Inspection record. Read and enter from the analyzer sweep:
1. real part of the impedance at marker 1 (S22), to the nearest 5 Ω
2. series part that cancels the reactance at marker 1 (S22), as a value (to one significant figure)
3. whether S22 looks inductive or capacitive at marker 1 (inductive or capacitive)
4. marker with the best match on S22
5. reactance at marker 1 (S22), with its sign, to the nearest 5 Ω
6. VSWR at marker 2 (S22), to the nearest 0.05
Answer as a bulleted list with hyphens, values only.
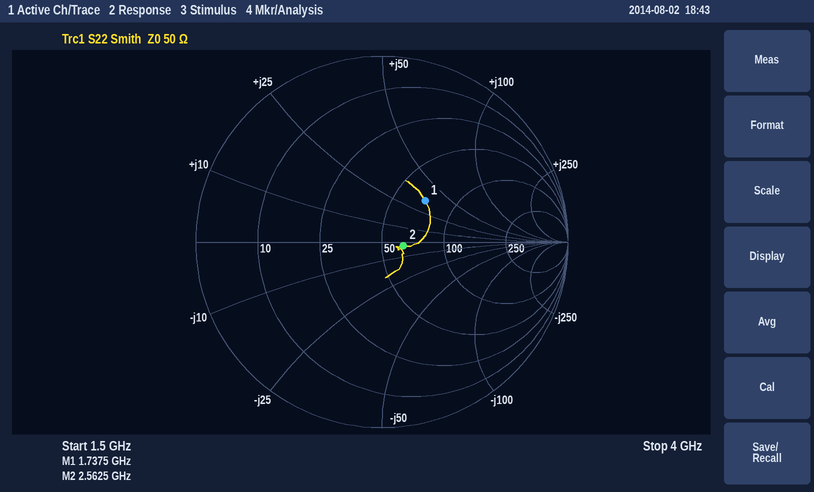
- 70 Ω
- 3 pF
- inductive
- marker 2
- +35 Ω
- 1.25
